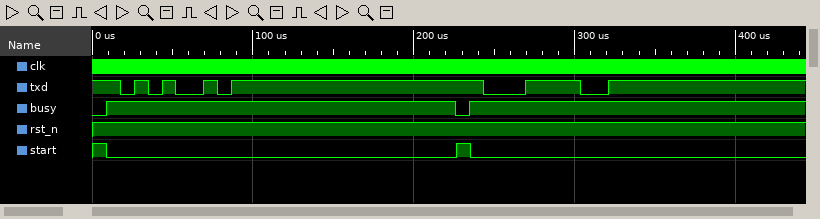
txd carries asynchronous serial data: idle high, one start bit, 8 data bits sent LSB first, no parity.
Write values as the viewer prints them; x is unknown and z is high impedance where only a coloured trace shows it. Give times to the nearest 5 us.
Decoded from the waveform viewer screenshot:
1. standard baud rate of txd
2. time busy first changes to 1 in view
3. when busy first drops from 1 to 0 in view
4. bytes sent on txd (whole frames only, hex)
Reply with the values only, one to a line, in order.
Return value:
115200 baud
10 us
225 us
A5, 3C
